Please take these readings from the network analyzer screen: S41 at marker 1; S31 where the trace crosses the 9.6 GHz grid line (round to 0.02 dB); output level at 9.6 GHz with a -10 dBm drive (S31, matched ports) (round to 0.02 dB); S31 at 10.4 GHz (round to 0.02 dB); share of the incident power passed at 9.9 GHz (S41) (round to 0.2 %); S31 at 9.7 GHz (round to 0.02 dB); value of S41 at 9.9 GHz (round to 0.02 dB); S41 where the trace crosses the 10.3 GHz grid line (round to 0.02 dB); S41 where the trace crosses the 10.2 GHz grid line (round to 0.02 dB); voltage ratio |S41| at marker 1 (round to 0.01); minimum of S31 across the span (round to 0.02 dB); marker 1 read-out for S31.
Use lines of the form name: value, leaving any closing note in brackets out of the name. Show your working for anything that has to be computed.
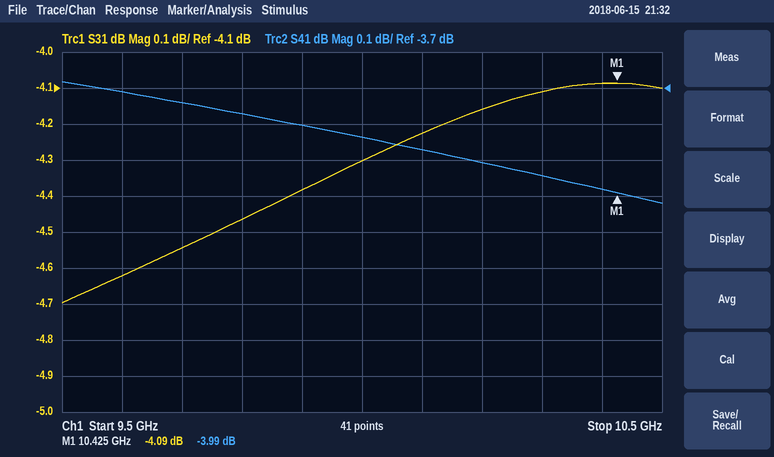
S41 at marker 1: -3.99 dB
S31 where the trace crosses the 9.6 GHz grid line: -4.62 dB
output level at 9.6 GHz with a -10 dBm drive (S31, matched ports): -10 dBm + (-4.62 dB) = -14.62 dBm
S31 at 10.4 GHz: -4.08 dB
share of the incident power passed at 9.9 GHz (S41): 10^(-3.8/10) ≈ 41.7 %, so 41.6 % to the nearest 0.2 %
S31 at 9.7 GHz: -4.54 dB
value of S41 at 9.9 GHz: -3.80 dB
S41 where the trace crosses the 10.3 GHz grid line: -3.94 dB
S41 where the trace crosses the 10.2 GHz grid line: -3.90 dB
voltage ratio |S41| at marker 1: 10^(-3.99/20) ≈ 0.63
minimum of S31 across the span: -4.70 dB
marker 1 read-out for S31: -4.09 dB
